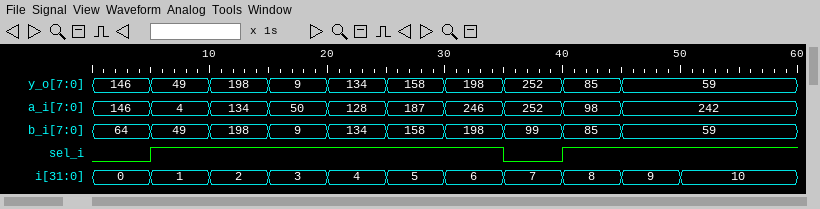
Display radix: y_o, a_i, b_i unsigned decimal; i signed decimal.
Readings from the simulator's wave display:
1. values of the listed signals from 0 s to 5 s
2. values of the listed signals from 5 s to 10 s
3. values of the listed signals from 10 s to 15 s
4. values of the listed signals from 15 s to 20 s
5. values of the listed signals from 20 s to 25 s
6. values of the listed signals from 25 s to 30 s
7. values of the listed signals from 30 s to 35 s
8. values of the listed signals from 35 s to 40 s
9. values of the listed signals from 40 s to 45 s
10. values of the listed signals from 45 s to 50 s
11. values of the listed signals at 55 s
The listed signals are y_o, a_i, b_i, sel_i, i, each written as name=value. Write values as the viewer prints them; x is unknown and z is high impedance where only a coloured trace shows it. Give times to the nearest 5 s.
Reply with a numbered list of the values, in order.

1. y_o=146, a_i=146, b_i=64, sel_i=0, i=0
2. y_o=49, a_i=4, b_i=49, sel_i=1, i=1
3. y_o=198, a_i=134, b_i=198, sel_i=1, i=2
4. y_o=9, a_i=50, b_i=9, sel_i=1, i=3
5. y_o=134, a_i=128, b_i=134, sel_i=1, i=4
6. y_o=158, a_i=187, b_i=158, sel_i=1, i=5
7. y_o=198, a_i=246, b_i=198, sel_i=1, i=6
8. y_o=252, a_i=252, b_i=99, sel_i=0, i=7
9. y_o=85, a_i=98, b_i=85, sel_i=1, i=8
10. y_o=59, a_i=242, b_i=59, sel_i=1, i=9
11. y_o=59, a_i=242, b_i=59, sel_i=1, i=10
